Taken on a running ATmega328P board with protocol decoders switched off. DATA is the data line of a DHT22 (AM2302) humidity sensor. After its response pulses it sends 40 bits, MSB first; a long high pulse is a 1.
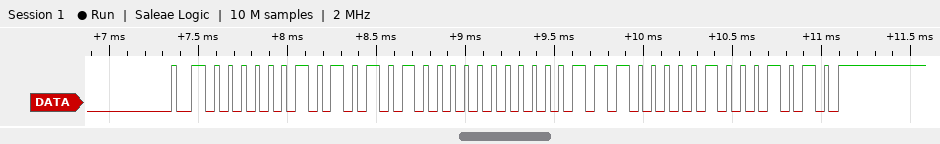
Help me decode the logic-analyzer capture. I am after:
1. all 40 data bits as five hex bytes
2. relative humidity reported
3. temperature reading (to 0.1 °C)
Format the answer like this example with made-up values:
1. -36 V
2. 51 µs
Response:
1. 02 A8 00 E0 8A
2. 68.0 %
3. 22.4 °C
